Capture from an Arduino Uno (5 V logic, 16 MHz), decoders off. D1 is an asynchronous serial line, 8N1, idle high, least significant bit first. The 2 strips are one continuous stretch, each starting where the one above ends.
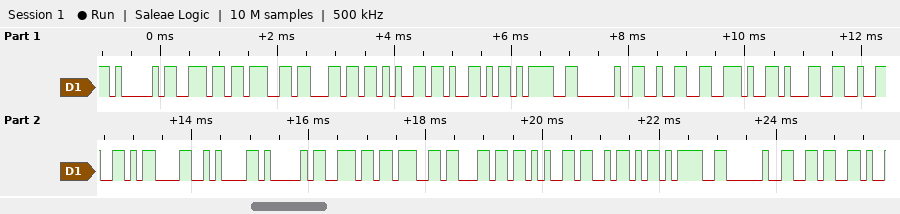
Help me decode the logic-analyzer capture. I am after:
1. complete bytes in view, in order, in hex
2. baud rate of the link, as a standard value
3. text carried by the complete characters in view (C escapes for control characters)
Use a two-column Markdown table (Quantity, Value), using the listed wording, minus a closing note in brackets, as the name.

| Quantity | Value |
|---|---|
| complete bytes in view, in order, in hex | 0x41 0x6E 0x67 0x6C 0x65 0x59 0x3D 0x20 0x32 0x2E 0x31 0x32 0x0D 0x0A 0x41 0x6E 0x67 0x6C 0x65 0x5A 0x3D 0x20 0x36 |
| baud rate of the link, as a standard value | 9600 baud |
| text carried by the complete characters in view | "AngleY= 2.12\r\nAngleZ= 6" |
